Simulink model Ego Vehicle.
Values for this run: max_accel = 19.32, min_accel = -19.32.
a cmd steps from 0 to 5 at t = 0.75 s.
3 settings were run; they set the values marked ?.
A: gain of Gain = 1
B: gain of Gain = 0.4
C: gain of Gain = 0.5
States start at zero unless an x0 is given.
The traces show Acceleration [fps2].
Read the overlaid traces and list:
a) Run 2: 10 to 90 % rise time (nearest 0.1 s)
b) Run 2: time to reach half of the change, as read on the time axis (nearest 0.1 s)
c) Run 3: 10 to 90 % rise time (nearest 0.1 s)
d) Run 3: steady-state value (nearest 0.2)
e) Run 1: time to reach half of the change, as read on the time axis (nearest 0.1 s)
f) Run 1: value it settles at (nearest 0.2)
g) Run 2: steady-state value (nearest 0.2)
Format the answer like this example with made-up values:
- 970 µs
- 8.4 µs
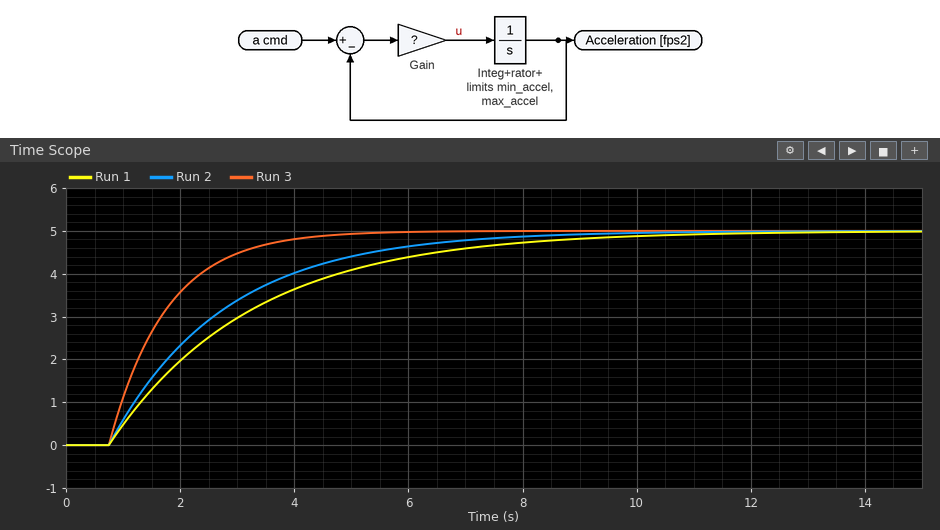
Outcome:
- 4.4 s
- 2.1 s
- 2.2 s
- 5.0
- 2.5 s
- 5.0
- 5.0
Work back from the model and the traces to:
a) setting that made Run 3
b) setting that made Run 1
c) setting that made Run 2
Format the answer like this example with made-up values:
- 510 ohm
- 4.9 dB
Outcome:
- A
- B
- C
